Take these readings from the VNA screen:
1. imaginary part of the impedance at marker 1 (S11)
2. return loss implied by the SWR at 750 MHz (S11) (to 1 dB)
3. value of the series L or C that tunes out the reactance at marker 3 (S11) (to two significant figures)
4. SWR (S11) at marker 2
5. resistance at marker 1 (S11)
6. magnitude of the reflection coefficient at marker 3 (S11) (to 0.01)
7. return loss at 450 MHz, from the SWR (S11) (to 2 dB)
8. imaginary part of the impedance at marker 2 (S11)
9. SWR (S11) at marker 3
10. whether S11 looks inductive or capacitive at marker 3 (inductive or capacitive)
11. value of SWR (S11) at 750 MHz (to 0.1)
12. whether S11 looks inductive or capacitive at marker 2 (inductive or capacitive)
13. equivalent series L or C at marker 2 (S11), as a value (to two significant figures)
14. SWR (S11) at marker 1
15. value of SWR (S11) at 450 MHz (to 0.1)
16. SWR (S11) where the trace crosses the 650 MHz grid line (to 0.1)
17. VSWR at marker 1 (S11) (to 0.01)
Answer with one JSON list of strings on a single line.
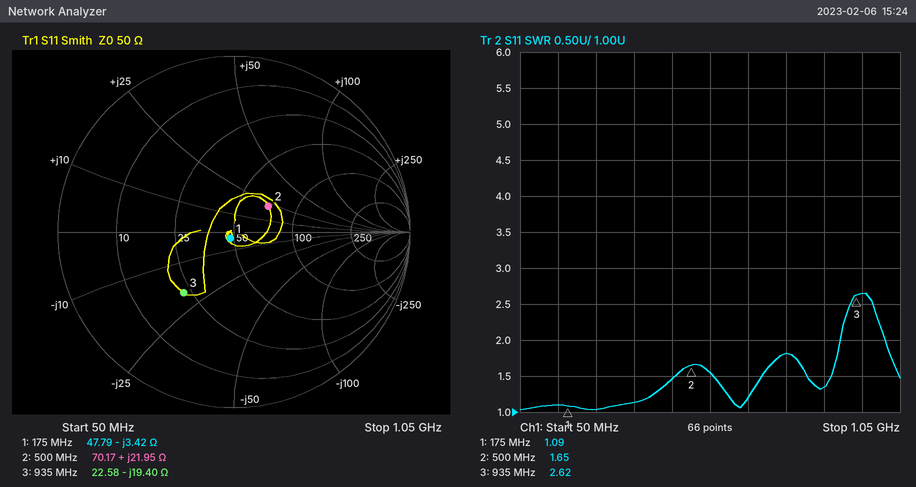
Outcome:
["-3.42 Ω", "11 dB", "3.3 nH", "1.65", "47.79 Ω", "0.45", "14 dB", "+21.95 Ω", "2.62", "capacitive", "1.8", "inductive", "7.0 nH", "1.09", "1.5", "1.2", "1.09"]
